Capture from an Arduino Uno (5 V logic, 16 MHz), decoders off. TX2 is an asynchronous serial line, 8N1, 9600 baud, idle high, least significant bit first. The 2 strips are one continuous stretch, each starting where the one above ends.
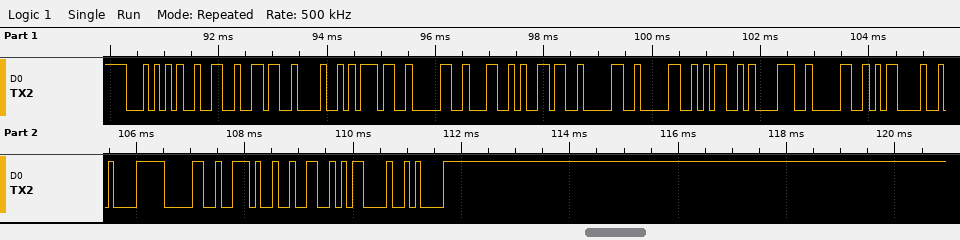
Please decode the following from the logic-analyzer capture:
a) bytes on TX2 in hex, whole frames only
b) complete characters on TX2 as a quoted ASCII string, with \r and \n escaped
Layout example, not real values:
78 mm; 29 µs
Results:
54 32 36 48 37 30 4C 36 30 30 4D 38 30 0D 0A 30 2E 32 0D 0A; "T26H70L600M80\r\n0.2\r\n"
